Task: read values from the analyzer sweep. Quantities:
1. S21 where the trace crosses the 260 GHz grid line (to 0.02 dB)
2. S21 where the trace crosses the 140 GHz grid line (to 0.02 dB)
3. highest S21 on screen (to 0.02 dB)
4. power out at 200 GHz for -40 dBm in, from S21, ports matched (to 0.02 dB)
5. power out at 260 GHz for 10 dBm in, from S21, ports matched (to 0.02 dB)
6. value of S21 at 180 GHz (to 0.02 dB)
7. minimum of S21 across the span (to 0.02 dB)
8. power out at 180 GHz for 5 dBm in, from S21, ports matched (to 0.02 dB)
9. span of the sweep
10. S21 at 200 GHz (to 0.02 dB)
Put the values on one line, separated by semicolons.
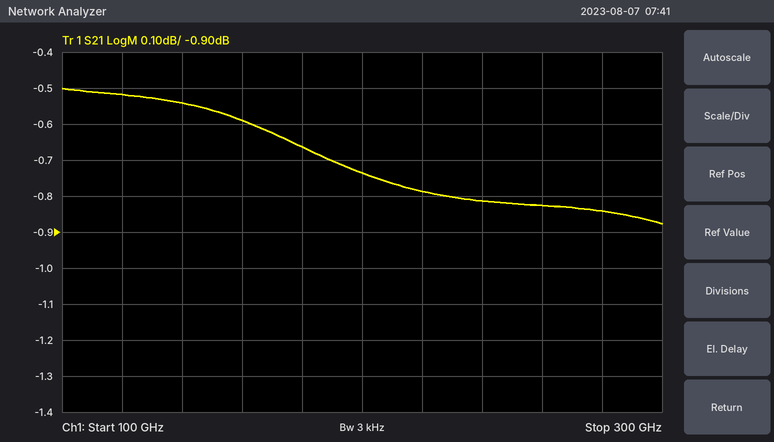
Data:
-0.82 dB; -0.54 dB; -0.50 dB; -40.74 dBm; 9.18 dBm; -0.66 dB; -0.88 dB; 4.34 dBm; 200 GHz; -0.74 dB
